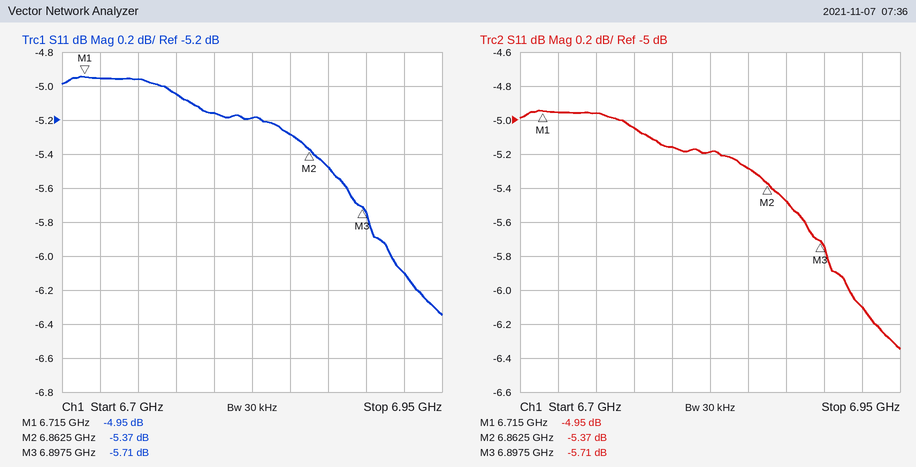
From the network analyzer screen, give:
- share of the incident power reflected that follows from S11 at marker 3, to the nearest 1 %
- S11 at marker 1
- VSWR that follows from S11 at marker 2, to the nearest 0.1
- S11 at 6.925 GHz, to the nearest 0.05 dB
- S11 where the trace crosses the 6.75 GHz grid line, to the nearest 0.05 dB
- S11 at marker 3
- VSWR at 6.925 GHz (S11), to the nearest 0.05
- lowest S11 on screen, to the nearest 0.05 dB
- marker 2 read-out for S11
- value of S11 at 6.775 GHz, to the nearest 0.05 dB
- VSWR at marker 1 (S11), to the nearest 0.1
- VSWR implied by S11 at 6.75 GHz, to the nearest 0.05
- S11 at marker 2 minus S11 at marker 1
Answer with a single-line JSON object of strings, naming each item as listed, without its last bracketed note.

{"share of the incident power reflected that follows from S11 at marker 3, to the nearest 1 %": "27 %", "S11 at marker 1": "-4.95 dB", "VSWR that follows from S11 at marker 2, to the nearest 0.1": "3.3", "S11 at 6.925 GHz, to the nearest 0.05 dB": "-6.10 dB", "S11 where the trace crosses the 6.75 GHz grid line, to the nearest 0.05 dB": "-4.95 dB", "S11 at marker 3": "-5.71 dB", "VSWR at 6.925 GHz (S11), to the nearest 0.05": "2.95", "lowest S11 on screen, to the nearest 0.05 dB": "-6.35 dB", "marker 2 read-out for S11": "-5.37 dB", "value of S11 at 6.775 GHz, to the nearest 0.05 dB": "-5.05 dB", "VSWR at marker 1 (S11), to the nearest 0.1": "3.6", "VSWR implied by S11 at 6.75 GHz, to the nearest 0.05": "3.60", "S11 at marker 2 minus S11 at marker 1": "-0.42 dB"}
